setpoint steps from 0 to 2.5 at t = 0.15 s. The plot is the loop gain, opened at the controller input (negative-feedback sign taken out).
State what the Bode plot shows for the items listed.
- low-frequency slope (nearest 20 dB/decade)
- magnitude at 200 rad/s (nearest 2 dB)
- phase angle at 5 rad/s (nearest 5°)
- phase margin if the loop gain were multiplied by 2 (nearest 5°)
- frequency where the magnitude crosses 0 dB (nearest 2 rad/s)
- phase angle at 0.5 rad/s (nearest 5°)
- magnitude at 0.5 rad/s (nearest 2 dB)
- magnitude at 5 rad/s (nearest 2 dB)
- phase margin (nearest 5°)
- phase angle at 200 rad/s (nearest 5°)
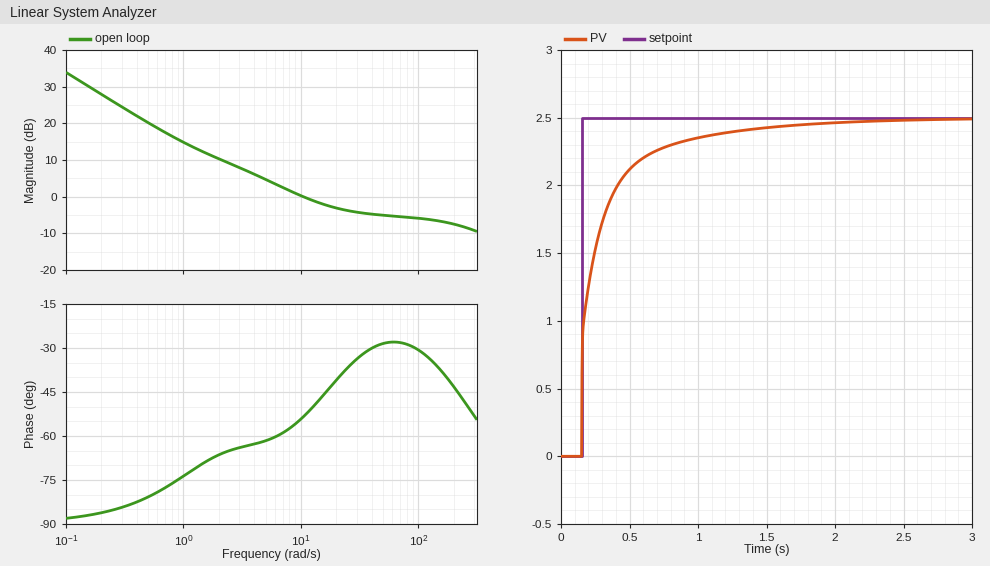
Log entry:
-20 dB/decade
-8 dB
-60°
150°
10 rad/s
-80°
20 dB
4 dB
125°
-45°
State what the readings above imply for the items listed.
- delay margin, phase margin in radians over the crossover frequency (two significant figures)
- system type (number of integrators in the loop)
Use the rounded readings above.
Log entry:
0.22 s
1
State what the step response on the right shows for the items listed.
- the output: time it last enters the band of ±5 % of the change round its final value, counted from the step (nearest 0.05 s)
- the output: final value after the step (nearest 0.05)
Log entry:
0.95 s
2.50
